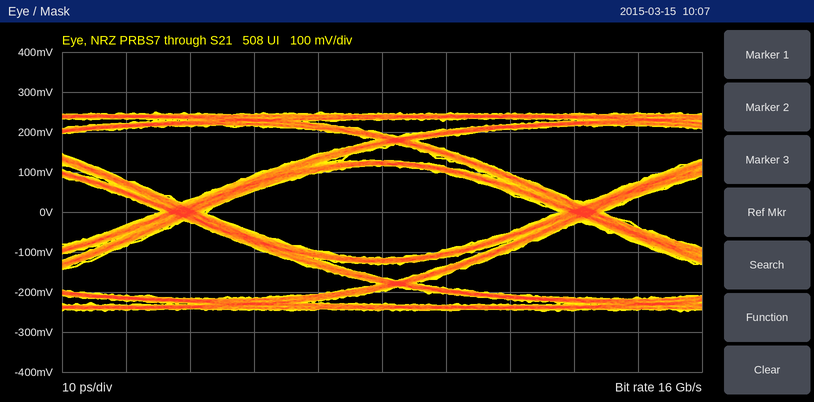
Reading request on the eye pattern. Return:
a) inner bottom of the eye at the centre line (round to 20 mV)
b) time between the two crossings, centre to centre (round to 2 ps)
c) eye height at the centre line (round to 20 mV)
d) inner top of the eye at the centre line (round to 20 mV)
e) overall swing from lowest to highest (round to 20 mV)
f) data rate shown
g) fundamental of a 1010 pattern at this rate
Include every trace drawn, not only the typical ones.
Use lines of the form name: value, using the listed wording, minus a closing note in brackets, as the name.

inner bottom of the eye at the centre line: -120 mV
time between the two crossings, centre to centre: 62 ps
eye height at the centre line: 240 mV
inner top of the eye at the centre line: 120 mV
overall swing from lowest to highest: 500 mV
data rate shown: 16 Gb/s
fundamental of a 1010 pattern at this rate: 8 GHz
